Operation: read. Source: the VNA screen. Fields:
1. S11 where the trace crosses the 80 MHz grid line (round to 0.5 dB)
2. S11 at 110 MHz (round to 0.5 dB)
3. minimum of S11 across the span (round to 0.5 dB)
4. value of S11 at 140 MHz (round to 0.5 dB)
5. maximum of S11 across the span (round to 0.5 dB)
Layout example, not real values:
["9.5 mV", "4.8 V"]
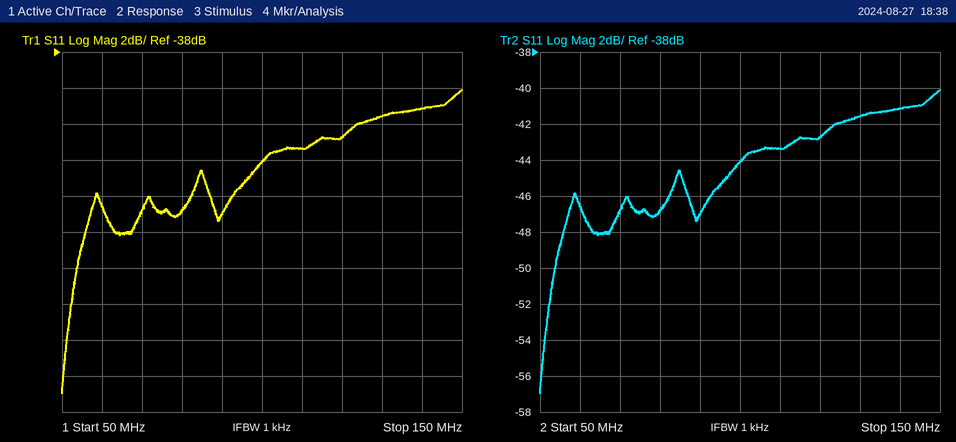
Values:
["-47.0 dB", "-43.5 dB", "-57.0 dB", "-41.0 dB", "-40.0 dB"]
